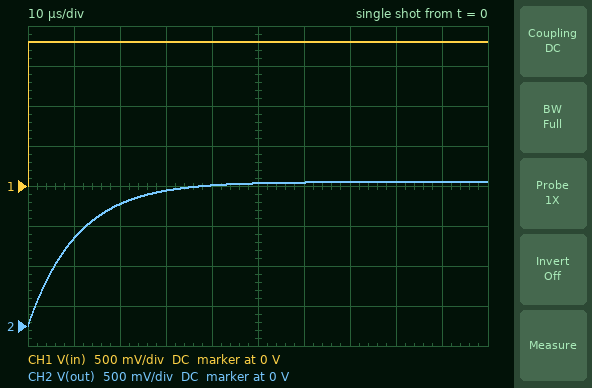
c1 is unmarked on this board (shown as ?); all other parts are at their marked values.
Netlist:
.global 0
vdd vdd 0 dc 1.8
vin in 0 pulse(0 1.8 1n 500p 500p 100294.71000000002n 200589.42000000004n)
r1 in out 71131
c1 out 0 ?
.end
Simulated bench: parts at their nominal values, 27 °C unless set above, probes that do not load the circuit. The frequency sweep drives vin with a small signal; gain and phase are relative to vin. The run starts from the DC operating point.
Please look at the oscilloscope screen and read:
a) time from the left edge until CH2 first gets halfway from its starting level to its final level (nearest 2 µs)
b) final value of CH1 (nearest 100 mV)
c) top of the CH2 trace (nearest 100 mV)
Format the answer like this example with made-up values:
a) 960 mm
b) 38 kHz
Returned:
a) 8 µs
b) 1.8 V
c) 1.8 V
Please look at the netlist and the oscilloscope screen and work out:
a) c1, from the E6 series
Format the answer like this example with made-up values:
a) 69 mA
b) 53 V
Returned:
a) 150 pF
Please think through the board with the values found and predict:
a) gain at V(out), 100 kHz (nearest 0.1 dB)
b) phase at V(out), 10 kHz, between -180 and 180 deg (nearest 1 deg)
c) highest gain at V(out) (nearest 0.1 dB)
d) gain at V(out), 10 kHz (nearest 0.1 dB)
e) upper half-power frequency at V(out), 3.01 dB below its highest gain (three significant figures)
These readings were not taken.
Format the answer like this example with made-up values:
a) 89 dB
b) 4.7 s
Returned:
a) -16.6 dB
b) -34 deg
c) 0 dB
d) -1.6 dB
e) 14.9 kHz
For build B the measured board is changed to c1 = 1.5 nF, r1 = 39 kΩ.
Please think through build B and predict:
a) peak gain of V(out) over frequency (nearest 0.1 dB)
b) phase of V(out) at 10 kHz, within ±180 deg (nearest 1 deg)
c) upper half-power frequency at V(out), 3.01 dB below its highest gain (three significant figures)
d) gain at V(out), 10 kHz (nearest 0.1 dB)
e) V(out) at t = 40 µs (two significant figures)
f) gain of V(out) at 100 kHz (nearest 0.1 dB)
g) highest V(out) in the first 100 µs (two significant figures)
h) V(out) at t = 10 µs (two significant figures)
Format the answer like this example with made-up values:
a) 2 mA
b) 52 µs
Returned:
a) 0 dB
b) -75 deg
c) 2.72 kHz
d) -11.6 dB
e) 890 mV
f) -31.3 dB
g) 1.5 V
h) 280 mV
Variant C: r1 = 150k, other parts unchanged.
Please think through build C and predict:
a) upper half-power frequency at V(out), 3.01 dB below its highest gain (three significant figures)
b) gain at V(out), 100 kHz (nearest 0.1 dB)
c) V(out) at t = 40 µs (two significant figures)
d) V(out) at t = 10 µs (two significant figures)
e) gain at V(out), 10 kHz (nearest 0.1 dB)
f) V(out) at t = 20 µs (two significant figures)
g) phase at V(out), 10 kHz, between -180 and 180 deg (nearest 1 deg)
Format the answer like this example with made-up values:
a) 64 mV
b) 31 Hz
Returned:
a) 7.07 kHz
b) -23.0 dB
c) 1.5 V
d) 650 mV
e) -4.8 dB
f) 1.1 V
g) -55 deg
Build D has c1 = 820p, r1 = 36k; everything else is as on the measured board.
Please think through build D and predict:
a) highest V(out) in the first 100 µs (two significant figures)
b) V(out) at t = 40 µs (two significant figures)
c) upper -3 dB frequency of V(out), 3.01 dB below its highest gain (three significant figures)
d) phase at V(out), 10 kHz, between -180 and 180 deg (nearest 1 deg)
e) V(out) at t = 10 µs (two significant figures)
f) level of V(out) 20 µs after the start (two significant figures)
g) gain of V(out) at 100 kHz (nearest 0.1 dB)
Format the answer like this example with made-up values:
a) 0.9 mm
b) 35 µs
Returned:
a) 1.7 V
b) 1.3 V
c) 5.39 kHz
d) -62 deg
e) 520 mV
f) 890 mV
g) -25.4 dB
